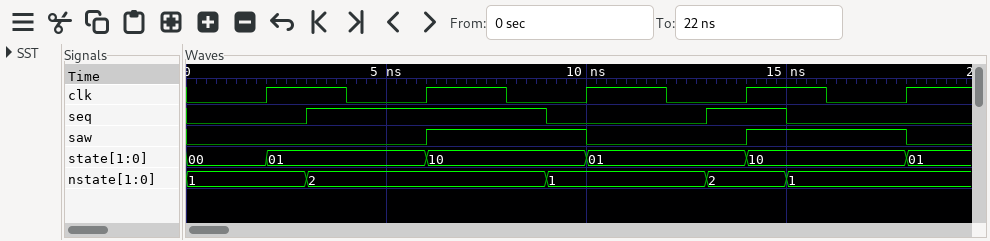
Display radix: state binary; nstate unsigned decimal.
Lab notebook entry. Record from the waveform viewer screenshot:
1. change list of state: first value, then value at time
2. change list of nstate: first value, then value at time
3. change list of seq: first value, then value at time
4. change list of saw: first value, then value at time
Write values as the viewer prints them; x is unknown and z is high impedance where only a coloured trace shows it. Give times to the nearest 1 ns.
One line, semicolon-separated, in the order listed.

00, 01 at 2 ns, 10 at 6 ns, 01 at 10 ns, 10 at 14 ns, 01 at 18 ns; 1, 2 at 3 ns, 1 at 9 ns, 2 at 13 ns, 1 at 15 ns; 0, 1 at 3 ns, 0 at 9 ns, 1 at 13 ns, 0 at 15 ns; 0, 1 at 6 ns, 0 at 10 ns, 1 at 14 ns, 0 at 18 ns
